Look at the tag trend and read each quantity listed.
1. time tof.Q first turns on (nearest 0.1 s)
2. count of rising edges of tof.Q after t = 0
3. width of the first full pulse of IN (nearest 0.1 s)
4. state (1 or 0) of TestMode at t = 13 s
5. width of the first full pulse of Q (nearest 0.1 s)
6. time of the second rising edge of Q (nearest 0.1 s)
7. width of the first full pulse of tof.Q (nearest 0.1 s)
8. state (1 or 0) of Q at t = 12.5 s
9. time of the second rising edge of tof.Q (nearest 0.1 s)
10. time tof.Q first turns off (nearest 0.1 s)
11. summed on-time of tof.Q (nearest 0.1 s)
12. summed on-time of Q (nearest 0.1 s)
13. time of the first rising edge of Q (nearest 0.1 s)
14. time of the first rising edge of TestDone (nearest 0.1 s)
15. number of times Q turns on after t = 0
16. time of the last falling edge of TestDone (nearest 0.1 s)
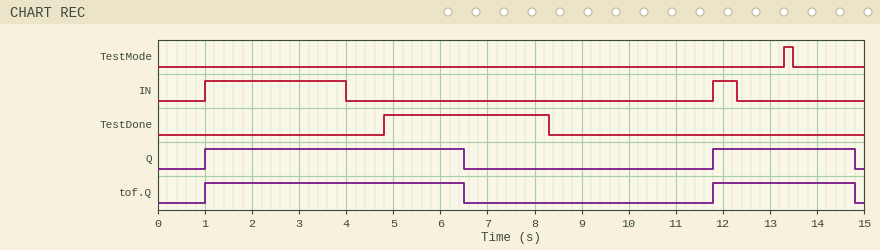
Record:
1.0 s
2
3.0 s
0
5.5 s
11.8 s
5.5 s
1
11.8 s
6.5 s
8.5 s
8.5 s
1.0 s
4.8 s
2
8.3 s
